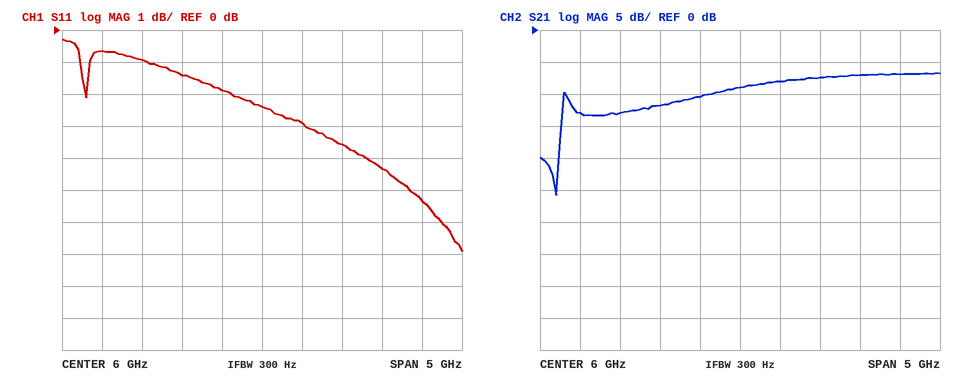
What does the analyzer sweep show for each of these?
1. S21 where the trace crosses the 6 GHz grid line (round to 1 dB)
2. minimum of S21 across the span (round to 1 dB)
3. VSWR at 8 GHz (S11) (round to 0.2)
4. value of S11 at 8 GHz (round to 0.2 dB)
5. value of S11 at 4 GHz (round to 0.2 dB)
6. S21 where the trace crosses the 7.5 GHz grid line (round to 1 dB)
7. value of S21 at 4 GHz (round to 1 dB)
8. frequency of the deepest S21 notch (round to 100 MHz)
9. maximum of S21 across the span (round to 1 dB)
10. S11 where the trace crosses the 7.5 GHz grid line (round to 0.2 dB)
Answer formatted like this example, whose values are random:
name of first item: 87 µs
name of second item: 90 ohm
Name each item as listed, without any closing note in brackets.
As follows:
S21 where the trace crosses the 6 GHz grid line: -9 dB
minimum of S21 across the span: -26 dB
VSWR at 8 GHz (S11): 3.4
value of S11 at 8 GHz: -5.4 dB
value of S11 at 4 GHz: -0.6 dB
S21 where the trace crosses the 7.5 GHz grid line: -7 dB
value of S21 at 4 GHz: -13 dB
frequency of the deepest S21 notch: 3.7 GHz
maximum of S21 across the span: -7 dB
S11 where the trace crosses the 7.5 GHz grid line: -4.4 dB
